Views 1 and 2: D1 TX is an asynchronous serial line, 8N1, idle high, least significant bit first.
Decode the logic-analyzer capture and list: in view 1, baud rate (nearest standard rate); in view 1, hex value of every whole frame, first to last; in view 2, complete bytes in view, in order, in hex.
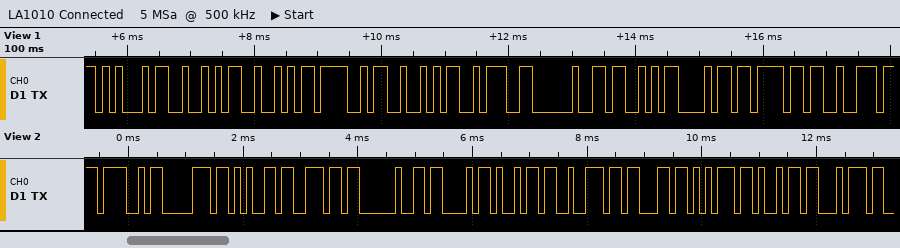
9600 baud
0x45 0x52 0x52 0x4F 0x52 0x3A 0x20 0x53 0x68 0x6F 0x72
4F 70 65 6E 20 43 69 72 63 75 69 74
